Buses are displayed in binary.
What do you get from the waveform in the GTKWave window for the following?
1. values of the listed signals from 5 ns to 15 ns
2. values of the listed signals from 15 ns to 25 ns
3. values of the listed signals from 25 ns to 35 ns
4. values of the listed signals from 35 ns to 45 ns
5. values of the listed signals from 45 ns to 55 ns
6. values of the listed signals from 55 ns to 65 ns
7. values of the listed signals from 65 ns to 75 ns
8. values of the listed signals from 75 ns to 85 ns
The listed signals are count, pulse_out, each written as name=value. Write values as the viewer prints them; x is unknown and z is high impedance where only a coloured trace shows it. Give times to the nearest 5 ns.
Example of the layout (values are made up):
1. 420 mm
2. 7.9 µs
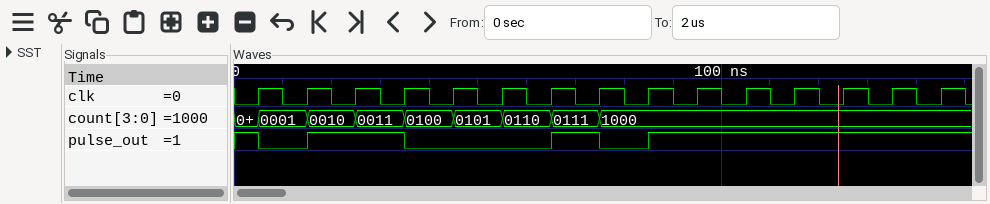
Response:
1. count=0001, pulse_out=0
2. count=0010, pulse_out=1
3. count=0011, pulse_out=1
4. count=0100, pulse_out=0
5. count=0101, pulse_out=0
6. count=0110, pulse_out=0
7. count=0111, pulse_out=1
8. count=1000, pulse_out=0
